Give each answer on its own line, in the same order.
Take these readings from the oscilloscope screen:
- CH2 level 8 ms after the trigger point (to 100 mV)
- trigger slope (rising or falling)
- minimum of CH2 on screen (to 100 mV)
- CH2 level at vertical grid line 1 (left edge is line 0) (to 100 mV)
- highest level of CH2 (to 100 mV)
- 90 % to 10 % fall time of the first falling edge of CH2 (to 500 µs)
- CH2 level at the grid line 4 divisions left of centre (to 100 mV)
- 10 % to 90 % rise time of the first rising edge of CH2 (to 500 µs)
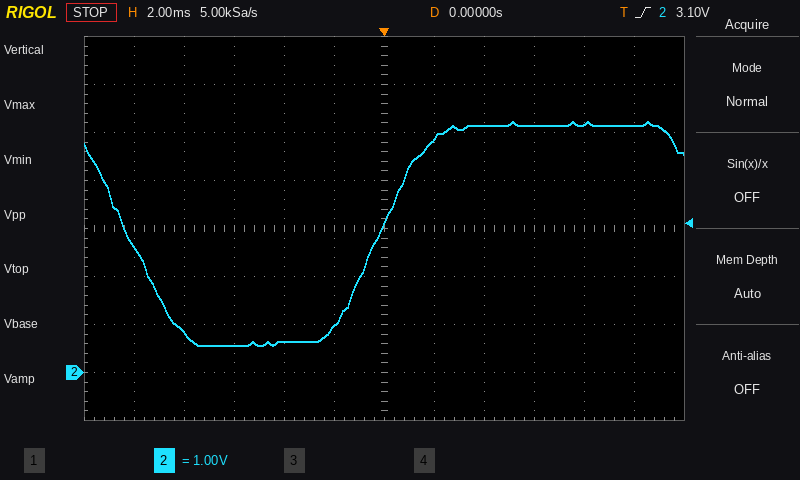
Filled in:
5.2 V
rising
600 mV
2.6 V
5.2 V
3.5 ms
800 mV
3.5 ms
